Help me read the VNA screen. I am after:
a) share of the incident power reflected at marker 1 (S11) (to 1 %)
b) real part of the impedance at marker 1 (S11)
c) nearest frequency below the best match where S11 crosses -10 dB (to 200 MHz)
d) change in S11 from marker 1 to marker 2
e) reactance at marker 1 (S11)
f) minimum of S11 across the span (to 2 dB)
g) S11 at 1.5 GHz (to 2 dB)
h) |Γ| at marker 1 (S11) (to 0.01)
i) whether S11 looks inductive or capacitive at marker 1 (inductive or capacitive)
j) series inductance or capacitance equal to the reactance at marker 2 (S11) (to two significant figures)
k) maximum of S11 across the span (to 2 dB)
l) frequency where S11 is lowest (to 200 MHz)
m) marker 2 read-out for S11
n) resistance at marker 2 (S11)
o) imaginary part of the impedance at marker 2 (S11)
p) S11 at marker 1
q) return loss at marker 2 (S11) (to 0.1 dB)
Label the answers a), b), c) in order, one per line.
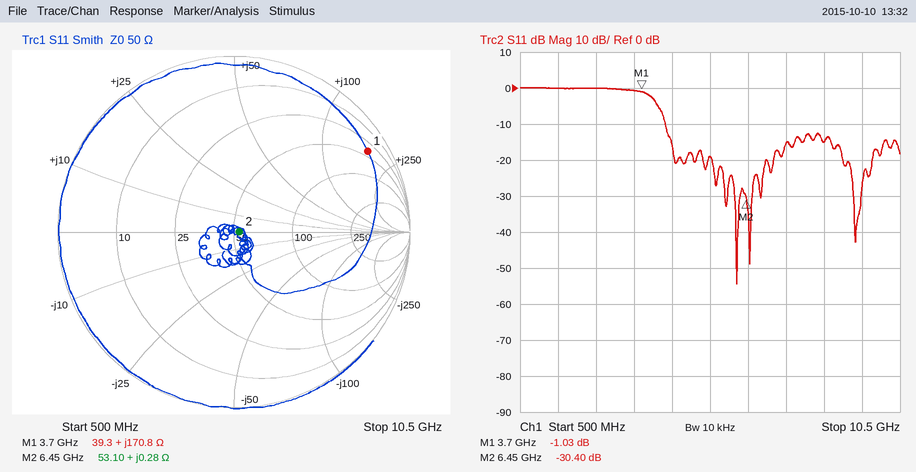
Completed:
a) 79 %
b) 39.3 Ω
c) 4.4 GHz
d) -29.37 dB
e) +170.8 Ω
f) -54 dB
g) 0 dB
h) 0.89
i) inductive
j) 6.9 pH
k) 0 dB
l) 6.2 GHz
m) -30.40 dB
n) 53.10 Ω
o) +0.28 Ω
p) -1.03 dB
q) 30.4 dB
